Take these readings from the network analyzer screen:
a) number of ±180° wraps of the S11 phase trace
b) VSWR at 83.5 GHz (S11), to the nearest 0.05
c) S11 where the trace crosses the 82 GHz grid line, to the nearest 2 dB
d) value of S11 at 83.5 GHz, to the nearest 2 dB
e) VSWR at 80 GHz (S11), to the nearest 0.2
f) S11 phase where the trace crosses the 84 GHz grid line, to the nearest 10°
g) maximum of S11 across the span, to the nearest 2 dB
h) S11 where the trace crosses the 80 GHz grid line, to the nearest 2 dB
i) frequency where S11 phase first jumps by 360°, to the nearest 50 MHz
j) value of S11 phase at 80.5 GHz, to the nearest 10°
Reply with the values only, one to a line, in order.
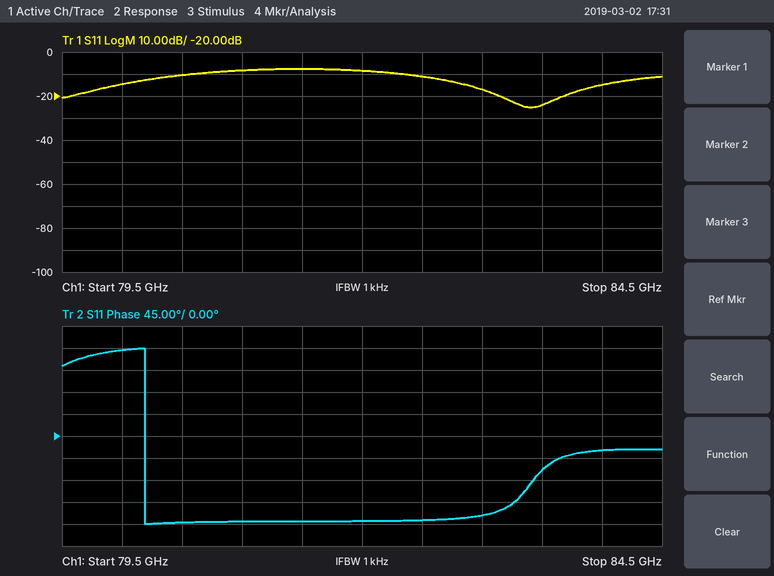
1
1.15
-8 dB
-24 dB
1.4
-30°
-8 dB
-14 dB
80.20 GHz
-180°
